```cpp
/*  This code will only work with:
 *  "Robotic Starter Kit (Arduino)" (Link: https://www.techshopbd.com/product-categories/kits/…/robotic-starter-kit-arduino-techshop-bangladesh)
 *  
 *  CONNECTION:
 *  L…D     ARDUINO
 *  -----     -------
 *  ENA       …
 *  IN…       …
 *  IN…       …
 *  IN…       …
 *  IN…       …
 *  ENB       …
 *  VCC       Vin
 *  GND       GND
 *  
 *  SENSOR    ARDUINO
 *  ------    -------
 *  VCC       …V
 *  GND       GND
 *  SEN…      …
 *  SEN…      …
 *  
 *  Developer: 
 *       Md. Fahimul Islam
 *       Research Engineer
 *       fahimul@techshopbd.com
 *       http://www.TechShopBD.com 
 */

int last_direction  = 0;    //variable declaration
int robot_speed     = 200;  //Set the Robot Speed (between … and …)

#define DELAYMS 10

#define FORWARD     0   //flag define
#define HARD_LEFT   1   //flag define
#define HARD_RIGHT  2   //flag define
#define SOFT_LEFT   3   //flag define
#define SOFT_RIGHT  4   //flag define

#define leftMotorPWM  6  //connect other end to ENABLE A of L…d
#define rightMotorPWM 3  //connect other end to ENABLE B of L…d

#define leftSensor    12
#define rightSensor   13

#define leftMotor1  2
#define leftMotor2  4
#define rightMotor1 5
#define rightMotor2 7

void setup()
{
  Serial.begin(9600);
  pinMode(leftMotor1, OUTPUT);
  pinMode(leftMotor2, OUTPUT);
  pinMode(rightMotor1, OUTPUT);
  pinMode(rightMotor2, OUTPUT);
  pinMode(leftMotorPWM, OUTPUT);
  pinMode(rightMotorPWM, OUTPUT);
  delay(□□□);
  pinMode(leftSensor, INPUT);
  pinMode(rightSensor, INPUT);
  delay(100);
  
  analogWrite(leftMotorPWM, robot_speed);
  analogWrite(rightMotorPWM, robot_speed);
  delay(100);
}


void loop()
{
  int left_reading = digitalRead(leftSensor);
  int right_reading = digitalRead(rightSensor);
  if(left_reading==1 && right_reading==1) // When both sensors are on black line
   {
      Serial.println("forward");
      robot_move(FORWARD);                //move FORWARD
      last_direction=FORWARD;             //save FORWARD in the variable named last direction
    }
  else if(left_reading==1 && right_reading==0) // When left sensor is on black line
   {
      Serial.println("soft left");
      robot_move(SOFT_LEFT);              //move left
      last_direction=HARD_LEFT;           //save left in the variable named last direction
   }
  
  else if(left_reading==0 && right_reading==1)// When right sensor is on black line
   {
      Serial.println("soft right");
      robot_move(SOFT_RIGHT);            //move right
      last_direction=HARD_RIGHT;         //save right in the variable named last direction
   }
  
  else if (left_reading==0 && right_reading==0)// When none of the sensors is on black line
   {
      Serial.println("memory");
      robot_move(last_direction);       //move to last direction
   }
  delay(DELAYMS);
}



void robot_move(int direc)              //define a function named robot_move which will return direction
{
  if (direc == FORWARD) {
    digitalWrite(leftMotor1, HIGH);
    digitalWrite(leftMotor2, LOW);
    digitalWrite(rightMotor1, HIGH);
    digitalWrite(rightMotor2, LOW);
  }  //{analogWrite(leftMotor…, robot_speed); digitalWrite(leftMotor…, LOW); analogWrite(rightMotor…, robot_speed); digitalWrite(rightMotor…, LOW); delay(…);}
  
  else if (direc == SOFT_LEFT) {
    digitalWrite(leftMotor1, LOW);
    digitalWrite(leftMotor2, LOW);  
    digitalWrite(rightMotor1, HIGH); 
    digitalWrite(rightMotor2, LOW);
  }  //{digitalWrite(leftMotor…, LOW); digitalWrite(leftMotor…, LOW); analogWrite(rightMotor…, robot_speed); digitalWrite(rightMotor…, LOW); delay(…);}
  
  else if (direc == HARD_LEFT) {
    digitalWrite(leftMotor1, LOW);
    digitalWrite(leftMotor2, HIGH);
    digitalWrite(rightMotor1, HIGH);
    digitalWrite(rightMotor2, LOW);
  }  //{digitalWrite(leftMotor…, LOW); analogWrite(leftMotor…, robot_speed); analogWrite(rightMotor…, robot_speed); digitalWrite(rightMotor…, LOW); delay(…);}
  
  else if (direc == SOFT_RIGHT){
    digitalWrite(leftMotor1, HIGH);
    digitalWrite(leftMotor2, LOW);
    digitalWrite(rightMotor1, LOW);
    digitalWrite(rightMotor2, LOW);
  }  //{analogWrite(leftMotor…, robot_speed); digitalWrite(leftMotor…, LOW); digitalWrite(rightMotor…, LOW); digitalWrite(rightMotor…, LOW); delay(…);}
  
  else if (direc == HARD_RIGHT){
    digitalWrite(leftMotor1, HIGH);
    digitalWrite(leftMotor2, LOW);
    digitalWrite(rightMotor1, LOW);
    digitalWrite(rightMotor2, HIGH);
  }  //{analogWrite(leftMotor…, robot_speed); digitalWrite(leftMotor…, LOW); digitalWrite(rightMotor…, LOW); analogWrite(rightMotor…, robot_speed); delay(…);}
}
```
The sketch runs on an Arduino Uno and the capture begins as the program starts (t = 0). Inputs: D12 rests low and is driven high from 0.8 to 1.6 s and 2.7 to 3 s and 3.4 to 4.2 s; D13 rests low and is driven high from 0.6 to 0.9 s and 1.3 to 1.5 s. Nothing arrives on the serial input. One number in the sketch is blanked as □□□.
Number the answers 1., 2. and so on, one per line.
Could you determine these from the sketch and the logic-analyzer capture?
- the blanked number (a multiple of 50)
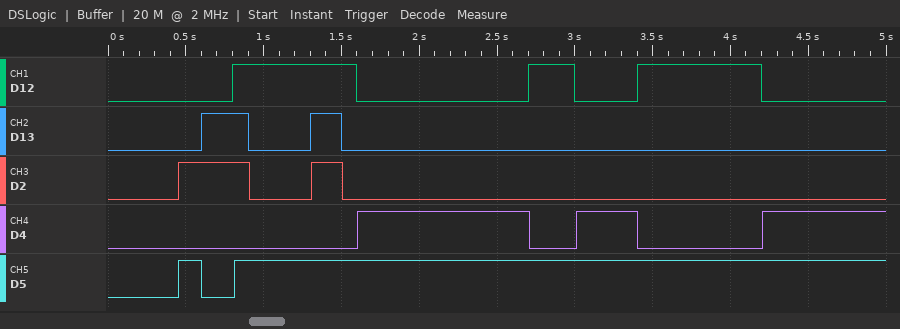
1. 250
